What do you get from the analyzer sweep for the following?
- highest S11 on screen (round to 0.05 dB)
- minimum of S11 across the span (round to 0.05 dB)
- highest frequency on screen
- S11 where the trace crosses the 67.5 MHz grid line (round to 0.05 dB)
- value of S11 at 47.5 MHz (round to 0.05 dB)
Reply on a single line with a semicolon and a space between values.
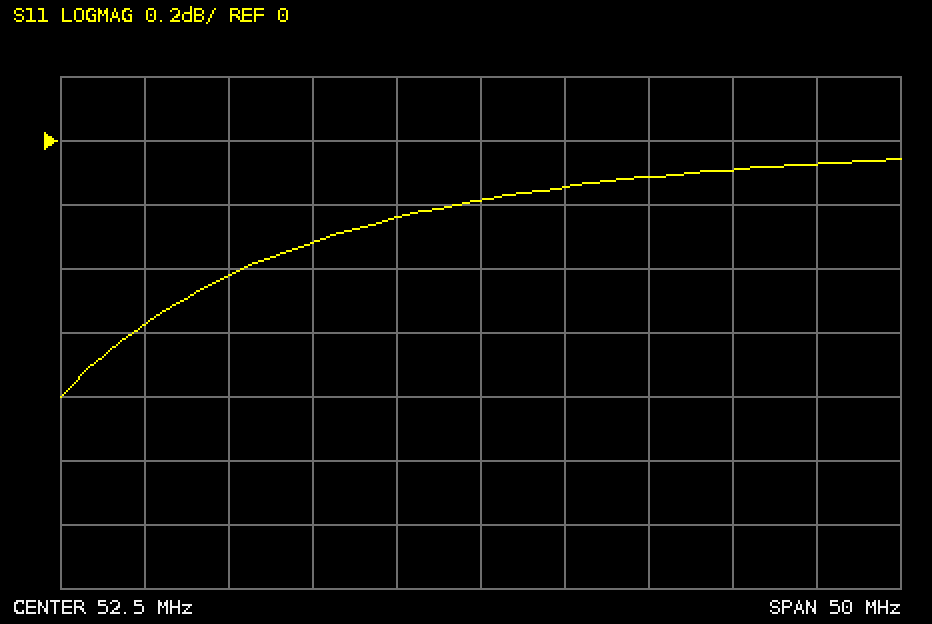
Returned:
-0.05 dB; -0.80 dB; 77.5 MHz; -0.10 dB; -0.25 dB
